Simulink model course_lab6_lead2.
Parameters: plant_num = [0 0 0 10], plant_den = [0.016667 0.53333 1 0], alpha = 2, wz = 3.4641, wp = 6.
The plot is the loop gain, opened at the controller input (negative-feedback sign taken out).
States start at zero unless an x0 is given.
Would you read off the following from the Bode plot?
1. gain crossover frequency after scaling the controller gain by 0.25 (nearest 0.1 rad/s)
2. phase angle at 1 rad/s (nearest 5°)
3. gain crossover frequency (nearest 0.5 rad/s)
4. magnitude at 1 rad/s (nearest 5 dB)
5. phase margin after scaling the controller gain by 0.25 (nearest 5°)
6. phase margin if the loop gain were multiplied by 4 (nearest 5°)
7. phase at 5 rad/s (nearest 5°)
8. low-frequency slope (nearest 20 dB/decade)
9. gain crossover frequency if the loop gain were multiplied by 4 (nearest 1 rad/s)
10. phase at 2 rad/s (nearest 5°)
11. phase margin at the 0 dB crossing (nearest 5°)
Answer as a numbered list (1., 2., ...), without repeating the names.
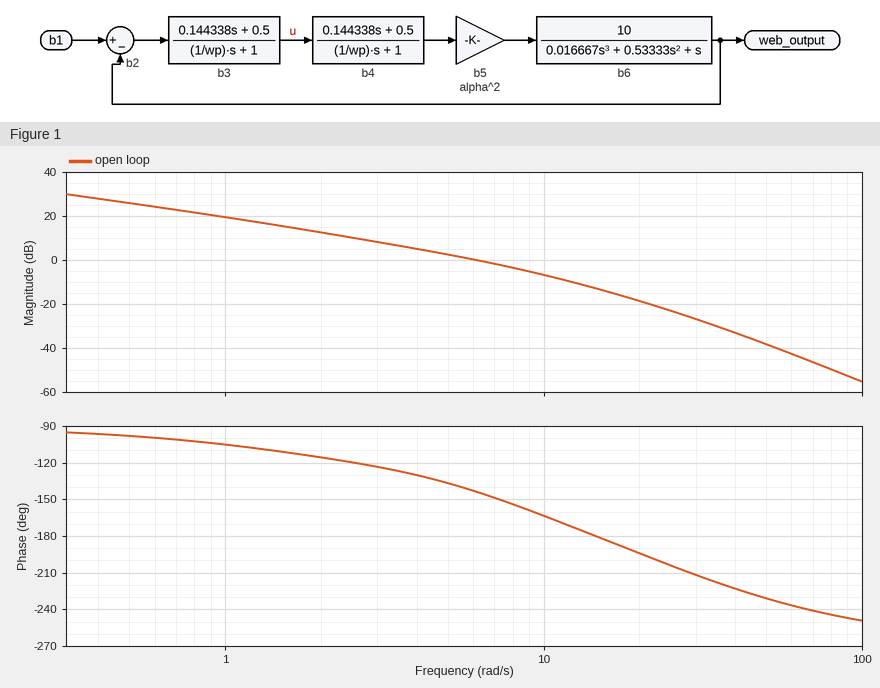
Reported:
1. 2.1 rad/s
2. -105°
3. 6.0 rad/s
4. 20 dB
5. 65°
6. 0°
7. -135°
8. -20 dB/decade
9. 14 rad/s
10. -115°
11. 35°
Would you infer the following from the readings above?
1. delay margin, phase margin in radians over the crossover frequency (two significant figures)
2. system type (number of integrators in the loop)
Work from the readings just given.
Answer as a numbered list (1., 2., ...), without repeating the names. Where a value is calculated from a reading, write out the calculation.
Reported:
1. 35 × π / 180 / 6 = 0.10 s
2. 1
